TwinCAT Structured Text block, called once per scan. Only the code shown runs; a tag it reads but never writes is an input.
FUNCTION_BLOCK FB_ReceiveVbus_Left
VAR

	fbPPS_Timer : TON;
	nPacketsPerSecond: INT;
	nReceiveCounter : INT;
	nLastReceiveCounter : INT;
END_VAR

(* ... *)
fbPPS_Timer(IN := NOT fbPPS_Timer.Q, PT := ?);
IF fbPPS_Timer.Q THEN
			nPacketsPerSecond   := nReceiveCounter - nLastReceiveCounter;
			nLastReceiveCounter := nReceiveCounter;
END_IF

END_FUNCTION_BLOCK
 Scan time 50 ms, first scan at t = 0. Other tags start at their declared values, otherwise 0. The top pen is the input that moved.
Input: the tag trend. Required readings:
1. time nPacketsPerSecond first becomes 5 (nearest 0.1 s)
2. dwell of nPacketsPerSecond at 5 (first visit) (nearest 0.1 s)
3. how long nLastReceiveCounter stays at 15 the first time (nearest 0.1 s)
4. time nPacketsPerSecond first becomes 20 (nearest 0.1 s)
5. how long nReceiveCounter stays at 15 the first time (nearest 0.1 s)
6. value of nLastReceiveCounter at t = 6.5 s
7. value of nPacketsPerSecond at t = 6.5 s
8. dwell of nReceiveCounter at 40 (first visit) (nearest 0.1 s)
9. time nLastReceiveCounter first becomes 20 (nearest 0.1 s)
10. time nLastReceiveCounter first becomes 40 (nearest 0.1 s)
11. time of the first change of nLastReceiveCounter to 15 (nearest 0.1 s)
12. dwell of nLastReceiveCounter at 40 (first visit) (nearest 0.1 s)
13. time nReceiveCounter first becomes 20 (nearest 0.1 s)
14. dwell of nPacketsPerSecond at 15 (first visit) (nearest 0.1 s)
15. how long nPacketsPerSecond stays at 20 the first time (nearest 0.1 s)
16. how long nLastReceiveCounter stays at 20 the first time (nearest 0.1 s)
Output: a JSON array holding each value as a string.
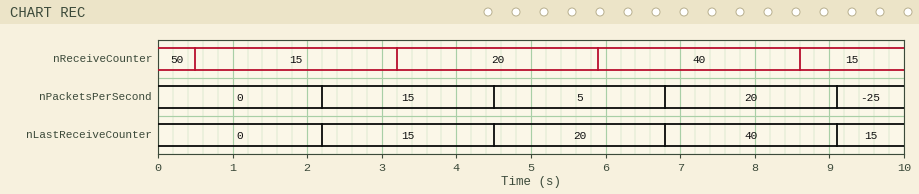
["4.5 s", "2.3 s", "2.3 s", "6.8 s", "2.7 s", "20", "5", "2.7 s", "4.5 s", "6.8 s", "2.2 s", "2.3 s", "3.2 s", "2.3 s", "2.3 s", "2.3 s"]
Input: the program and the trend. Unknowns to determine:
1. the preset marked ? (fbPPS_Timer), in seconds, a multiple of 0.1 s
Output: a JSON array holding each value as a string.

["2.2 s"]
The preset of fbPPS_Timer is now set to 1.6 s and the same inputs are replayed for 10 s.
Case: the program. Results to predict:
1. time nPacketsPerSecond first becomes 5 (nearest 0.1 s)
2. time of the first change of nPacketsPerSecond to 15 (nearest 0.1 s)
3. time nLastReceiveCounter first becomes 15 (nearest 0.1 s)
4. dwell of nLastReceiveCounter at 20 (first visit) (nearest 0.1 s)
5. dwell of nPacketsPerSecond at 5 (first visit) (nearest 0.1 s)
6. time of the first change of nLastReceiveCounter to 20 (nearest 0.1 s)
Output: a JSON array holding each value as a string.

["3.3 s", "1.6 s", "1.6 s", "3.4 s", "1.7 s", "3.3 s"]
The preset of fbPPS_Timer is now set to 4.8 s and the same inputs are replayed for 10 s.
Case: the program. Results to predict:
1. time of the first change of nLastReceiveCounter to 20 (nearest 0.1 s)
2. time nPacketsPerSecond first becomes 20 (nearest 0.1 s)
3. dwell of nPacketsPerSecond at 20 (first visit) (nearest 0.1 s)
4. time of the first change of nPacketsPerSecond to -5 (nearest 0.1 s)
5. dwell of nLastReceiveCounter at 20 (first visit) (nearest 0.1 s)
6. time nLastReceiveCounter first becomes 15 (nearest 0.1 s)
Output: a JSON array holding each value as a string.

["4.8 s", "4.8 s", "4.9 s", "9.7 s", "4.9 s", "9.7 s"]
